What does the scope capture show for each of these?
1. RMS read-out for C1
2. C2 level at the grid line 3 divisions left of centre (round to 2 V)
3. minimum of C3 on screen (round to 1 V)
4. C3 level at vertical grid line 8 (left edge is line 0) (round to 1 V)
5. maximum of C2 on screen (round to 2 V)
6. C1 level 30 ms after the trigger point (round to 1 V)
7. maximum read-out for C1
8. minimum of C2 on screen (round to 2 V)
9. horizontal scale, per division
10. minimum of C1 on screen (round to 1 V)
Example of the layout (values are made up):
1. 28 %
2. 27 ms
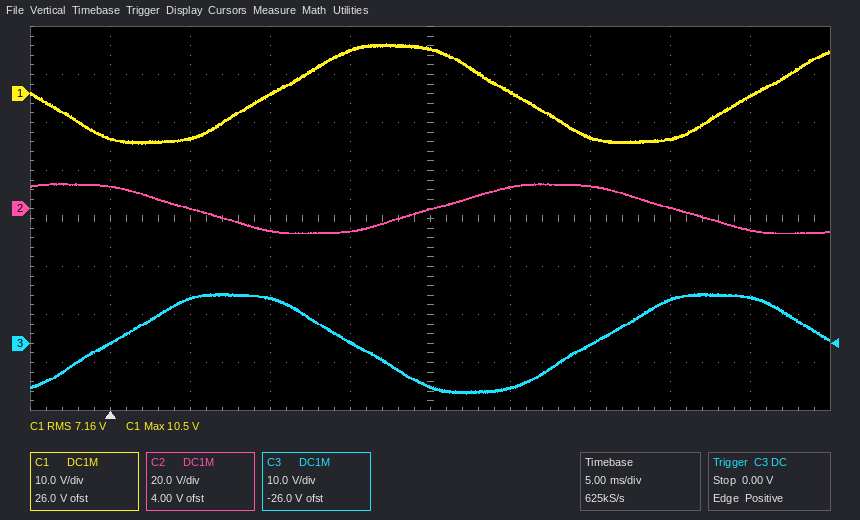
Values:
1. 7.16 V
2. 0 V
3. -11 V
4. 9 V
5. 10 V
6. -9 V
7. 10.5 V
8. -10 V
9. 5 ms
10. -11 V
